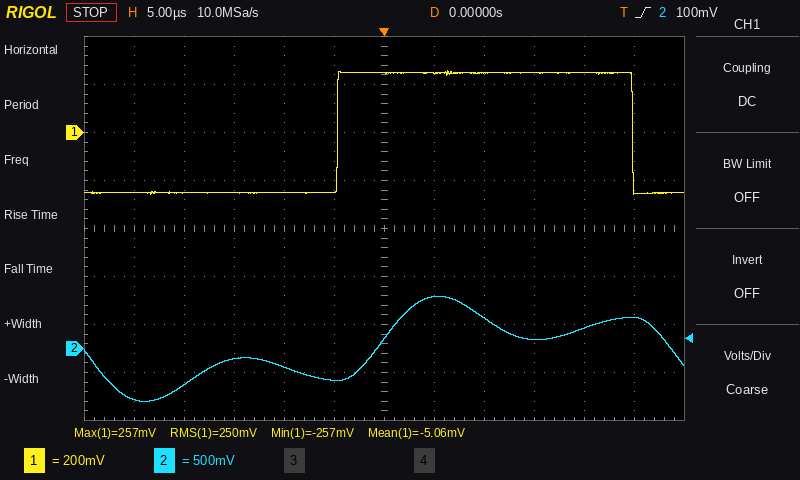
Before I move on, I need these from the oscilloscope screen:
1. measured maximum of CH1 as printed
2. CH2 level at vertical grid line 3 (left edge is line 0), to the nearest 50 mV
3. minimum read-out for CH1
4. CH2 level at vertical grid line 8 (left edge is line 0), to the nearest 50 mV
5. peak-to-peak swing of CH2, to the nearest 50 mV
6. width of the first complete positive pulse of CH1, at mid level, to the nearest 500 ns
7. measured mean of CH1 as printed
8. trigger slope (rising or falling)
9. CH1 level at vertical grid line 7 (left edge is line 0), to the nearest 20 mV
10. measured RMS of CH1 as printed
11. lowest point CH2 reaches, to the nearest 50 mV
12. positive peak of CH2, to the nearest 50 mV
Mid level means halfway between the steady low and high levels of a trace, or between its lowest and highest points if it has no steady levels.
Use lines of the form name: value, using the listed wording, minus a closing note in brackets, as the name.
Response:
measured maximum of CH1 as printed: 257 mV
CH2 level at vertical grid line 3 (left edge is line 0), to the nearest 50 mV: -100 mV
minimum read-out for CH1: -257 mV
CH2 level at vertical grid line 8 (left edge is line 0), to the nearest 50 mV: 300 mV
peak-to-peak swing of CH2, to the nearest 50 mV: 1.10 V
width of the first complete positive pulse of CH1, at mid level, to the nearest 500 ns: 29.5 µs
measured mean of CH1 as printed: -5.06 mV
trigger slope: rising
CH1 level at vertical grid line 7 (left edge is line 0), to the nearest 20 mV: 240 mV
measured RMS of CH1 as printed: 250 mV
lowest point CH2 reaches, to the nearest 50 mV: -550 mV
positive peak of CH2, to the nearest 50 mV: 550 mV
